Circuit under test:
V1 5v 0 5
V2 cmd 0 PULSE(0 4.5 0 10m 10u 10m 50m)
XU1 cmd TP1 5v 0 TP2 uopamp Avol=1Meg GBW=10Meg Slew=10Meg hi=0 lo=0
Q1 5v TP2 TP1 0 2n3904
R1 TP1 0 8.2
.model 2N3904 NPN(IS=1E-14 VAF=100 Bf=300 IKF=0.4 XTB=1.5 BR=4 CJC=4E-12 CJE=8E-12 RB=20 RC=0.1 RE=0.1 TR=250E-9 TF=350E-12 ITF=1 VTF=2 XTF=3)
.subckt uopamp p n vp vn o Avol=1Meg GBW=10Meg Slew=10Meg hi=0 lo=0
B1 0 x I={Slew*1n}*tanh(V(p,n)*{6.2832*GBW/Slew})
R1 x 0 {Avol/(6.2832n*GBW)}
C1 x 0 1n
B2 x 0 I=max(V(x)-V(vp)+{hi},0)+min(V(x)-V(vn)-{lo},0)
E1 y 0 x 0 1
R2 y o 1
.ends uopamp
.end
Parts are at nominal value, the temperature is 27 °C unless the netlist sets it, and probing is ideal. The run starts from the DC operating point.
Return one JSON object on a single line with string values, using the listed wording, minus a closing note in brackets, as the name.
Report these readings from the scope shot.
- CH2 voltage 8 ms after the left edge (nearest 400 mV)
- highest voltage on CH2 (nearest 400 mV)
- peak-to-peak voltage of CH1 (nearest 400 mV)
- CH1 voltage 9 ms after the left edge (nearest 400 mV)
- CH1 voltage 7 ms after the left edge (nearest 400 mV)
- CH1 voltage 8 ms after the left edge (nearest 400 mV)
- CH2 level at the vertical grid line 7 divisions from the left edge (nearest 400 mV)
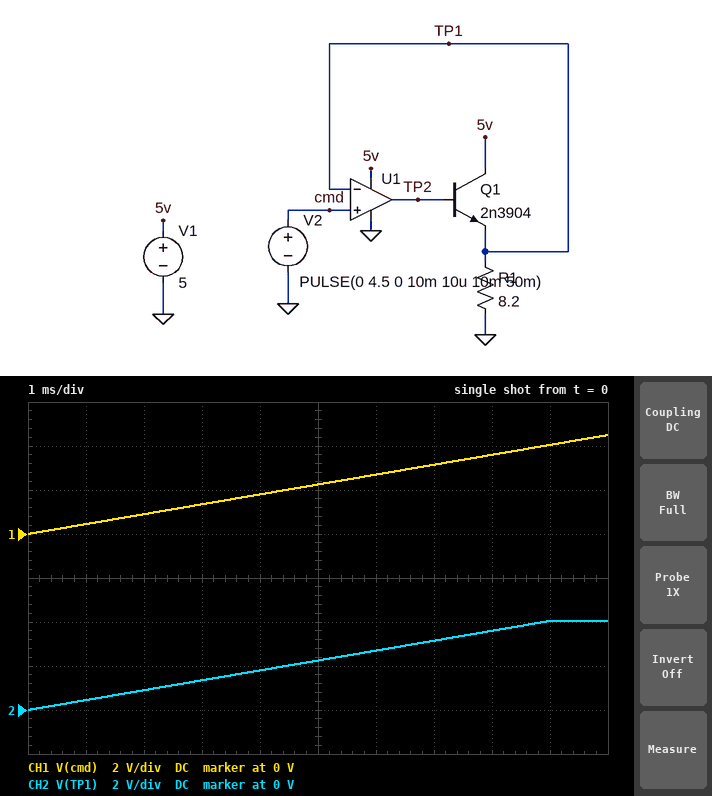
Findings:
{"CH2 voltage 8 ms after the left edge": "3.6 V", "highest voltage on CH2": "4.0 V", "peak-to-peak voltage of CH1": "4.4 V", "CH1 voltage 9 ms after the left edge": "4.0 V", "CH1 voltage 7 ms after the left edge": "3.2 V", "CH1 voltage 8 ms after the left edge": "3.6 V", "CH2 level at the vertical grid line 7 divisions from the left edge": "3.2 V"}
